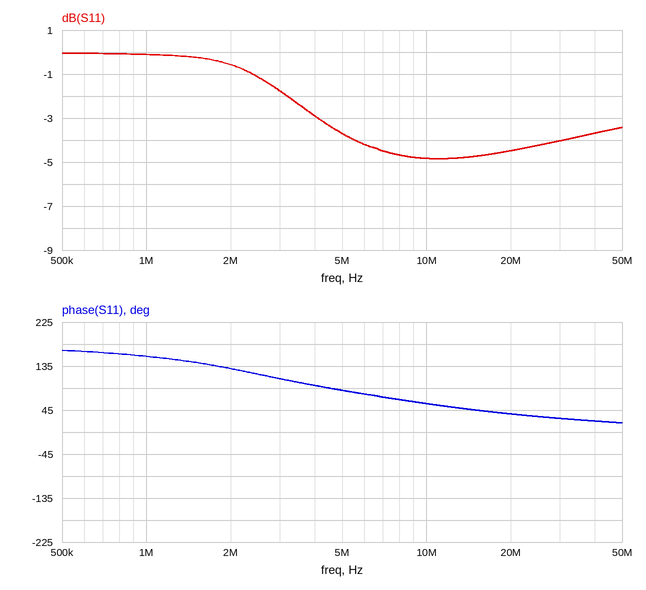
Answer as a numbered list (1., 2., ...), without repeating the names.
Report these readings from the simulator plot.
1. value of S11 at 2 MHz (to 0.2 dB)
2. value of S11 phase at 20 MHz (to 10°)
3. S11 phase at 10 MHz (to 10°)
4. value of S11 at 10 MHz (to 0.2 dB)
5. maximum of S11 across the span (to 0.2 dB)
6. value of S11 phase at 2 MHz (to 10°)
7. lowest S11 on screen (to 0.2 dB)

1. -0.6 dB
2. 40°
3. 60°
4. -4.8 dB
5. 0.0 dB
6. 130°
7. -4.8 dB
